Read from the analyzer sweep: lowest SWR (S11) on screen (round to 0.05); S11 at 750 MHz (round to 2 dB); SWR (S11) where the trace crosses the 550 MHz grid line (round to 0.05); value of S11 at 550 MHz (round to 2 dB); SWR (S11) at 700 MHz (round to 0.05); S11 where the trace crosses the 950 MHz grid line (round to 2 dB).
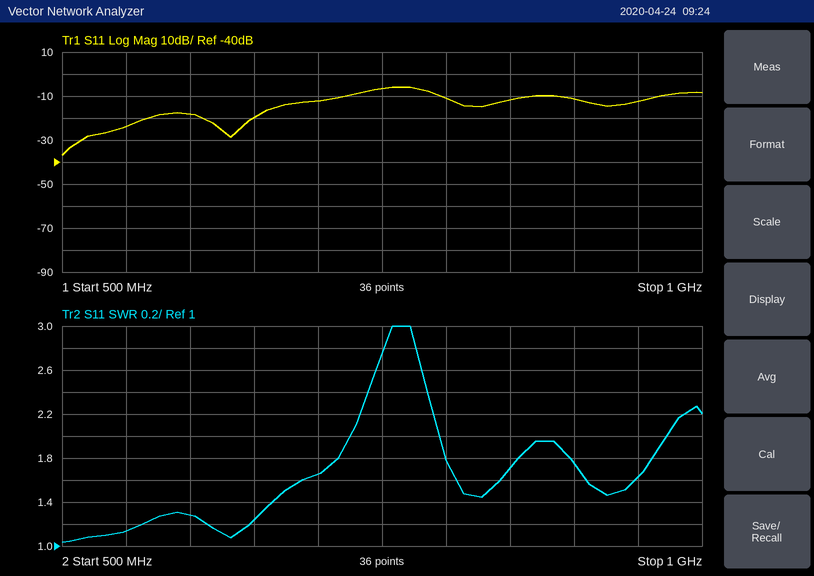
1.05
-6 dB
1.15
-24 dB
1.65
-12 dB
